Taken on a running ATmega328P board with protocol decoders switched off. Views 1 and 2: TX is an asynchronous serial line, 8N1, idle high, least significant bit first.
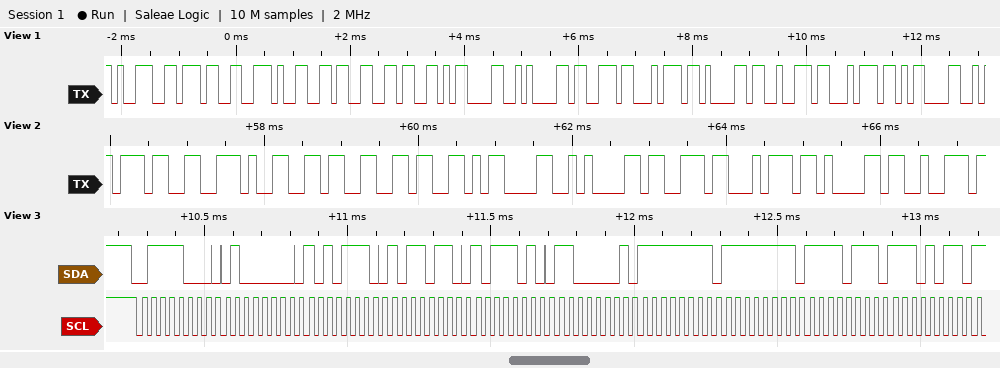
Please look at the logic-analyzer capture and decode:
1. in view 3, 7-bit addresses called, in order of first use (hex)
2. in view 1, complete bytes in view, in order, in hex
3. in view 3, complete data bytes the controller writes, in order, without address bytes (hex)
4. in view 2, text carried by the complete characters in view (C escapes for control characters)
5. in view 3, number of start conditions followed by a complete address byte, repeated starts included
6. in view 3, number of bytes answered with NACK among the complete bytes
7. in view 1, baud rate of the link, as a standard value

0x3C
39 37 2E 36 36 0D 0A 73 74 61 72 74 0D
40 AE B6 BA C1 FF FF F7 EB
"7.66\r\nstar"
1
0
9600 baud
